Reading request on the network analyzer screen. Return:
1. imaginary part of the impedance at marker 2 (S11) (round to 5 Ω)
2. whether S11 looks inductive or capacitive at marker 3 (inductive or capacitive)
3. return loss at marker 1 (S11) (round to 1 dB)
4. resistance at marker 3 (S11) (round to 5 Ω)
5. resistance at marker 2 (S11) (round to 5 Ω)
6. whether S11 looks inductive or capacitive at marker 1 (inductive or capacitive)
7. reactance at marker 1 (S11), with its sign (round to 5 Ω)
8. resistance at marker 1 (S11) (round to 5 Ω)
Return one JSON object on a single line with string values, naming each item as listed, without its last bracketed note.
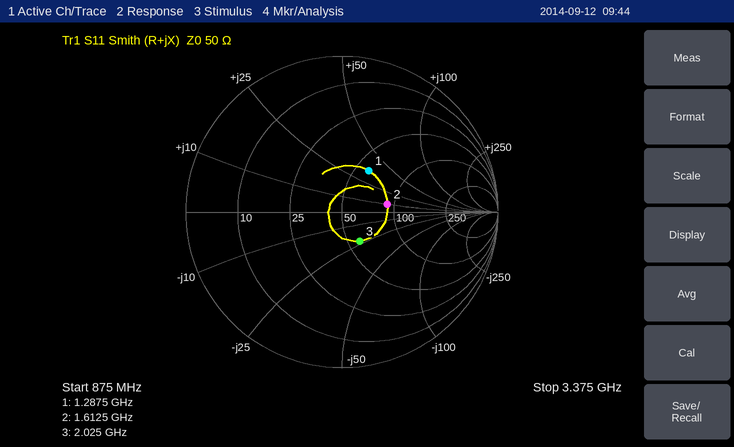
{"imaginary part of the impedance at marker 2 (S11)": "+10 Ω", "whether S11 looks inductive or capacitive at marker 3": "capacitive", "return loss at marker 1 (S11)": "10 dB", "resistance at marker 3 (S11)": "60 Ω", "resistance at marker 2 (S11)": "90 Ω", "whether S11 looks inductive or capacitive at marker 1": "inductive", "reactance at marker 1 (S11), with its sign": "+35 Ω", "resistance at marker 1 (S11)": "60 Ω"}
